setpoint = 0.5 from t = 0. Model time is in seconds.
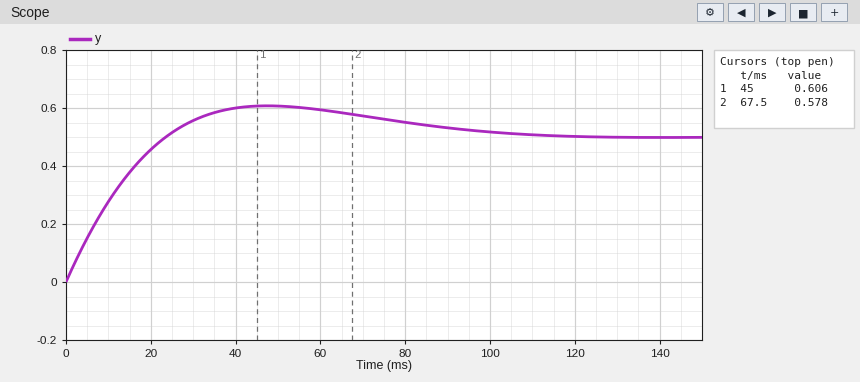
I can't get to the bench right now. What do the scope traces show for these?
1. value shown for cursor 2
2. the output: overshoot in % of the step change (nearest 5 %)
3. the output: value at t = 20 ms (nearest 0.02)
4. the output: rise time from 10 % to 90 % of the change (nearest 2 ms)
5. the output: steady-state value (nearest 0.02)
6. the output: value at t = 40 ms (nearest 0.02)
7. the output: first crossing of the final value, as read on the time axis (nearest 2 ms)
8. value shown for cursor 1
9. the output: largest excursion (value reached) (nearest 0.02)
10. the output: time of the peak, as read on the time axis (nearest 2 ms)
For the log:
0.578
20 %
0.46
18 ms
0.50
0.60
24 ms
0.606
0.60
48 ms
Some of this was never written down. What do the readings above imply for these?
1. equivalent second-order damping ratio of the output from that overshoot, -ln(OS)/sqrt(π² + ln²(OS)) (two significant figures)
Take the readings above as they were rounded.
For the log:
0.46
